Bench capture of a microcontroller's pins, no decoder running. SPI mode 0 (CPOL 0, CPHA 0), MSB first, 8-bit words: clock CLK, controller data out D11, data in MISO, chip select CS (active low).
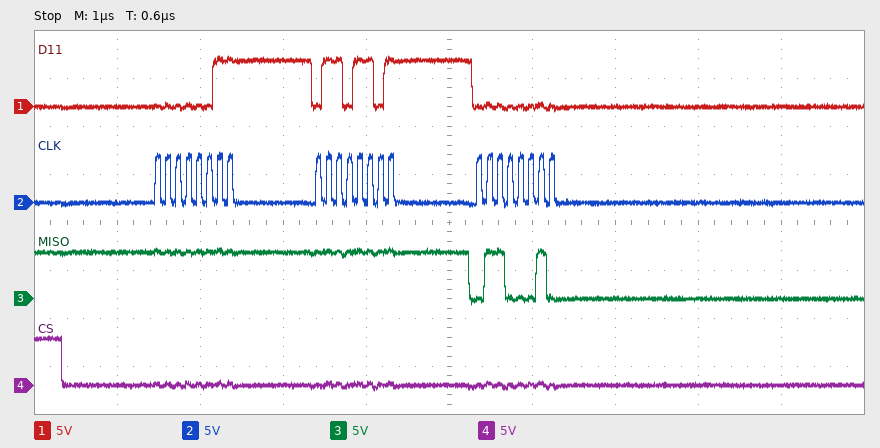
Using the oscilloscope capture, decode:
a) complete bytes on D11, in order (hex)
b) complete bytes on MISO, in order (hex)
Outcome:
03 6D 00
FF FF 62
